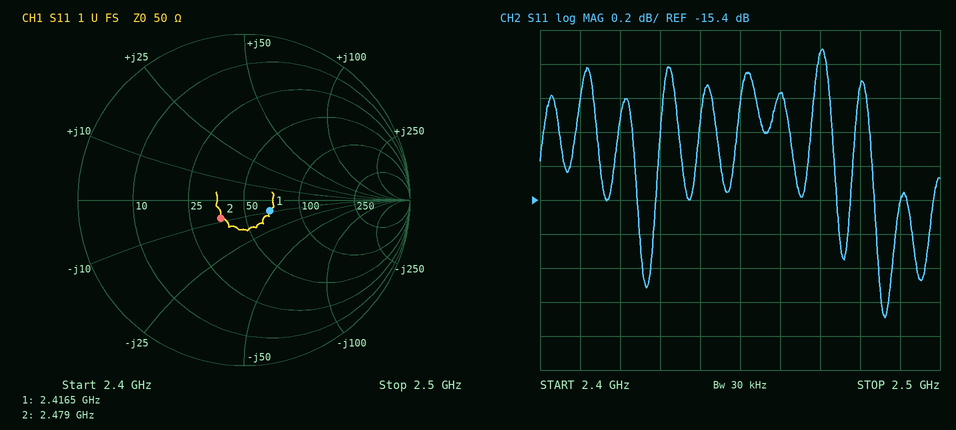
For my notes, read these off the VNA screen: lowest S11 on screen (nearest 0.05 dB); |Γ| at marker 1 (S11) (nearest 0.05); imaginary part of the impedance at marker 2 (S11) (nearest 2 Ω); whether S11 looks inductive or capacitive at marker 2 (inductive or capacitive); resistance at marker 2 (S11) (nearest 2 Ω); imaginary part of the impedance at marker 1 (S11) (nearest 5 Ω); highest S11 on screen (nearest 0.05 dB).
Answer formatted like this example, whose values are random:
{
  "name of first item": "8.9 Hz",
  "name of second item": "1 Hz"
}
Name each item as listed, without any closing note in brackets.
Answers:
{
  "lowest S11 on screen": "-16.10 dB",
  "|Γ| at marker 1 (S11)": "0.15",
  "imaginary part of the impedance at marker 2 (S11)": "-8 Ω",
  "whether S11 looks inductive or capacitive at marker 2": "capacitive",
  "resistance at marker 2 (S11)": "36 Ω",
  "imaginary part of the impedance at marker 1 (S11)": "-10 Ω",
  "highest S11 on screen": "-14.50 dB"
}
